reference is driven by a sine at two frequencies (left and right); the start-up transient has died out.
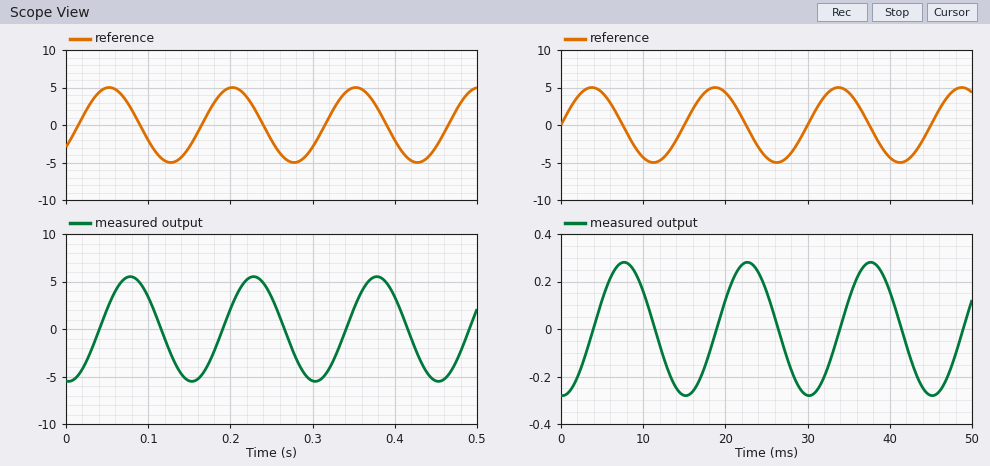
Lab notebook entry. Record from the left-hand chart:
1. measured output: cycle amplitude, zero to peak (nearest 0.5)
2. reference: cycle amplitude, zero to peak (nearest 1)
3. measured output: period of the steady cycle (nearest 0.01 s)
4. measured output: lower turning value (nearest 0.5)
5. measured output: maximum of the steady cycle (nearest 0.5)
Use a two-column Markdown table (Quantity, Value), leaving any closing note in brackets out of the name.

| Quantity | Value |
|---|---|
| measured output: cycle amplitude, zero to peak | 5.5 |
| reference: cycle amplitude, zero to peak | 5 |
| measured output: period of the steady cycle | 0.15 s |
| measured output: lower turning value | -5.5 |
| measured output: maximum of the steady cycle | 5.5 |
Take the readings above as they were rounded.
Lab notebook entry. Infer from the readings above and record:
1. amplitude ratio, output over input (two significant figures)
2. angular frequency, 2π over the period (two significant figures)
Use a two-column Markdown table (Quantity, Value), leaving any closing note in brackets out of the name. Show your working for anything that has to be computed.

| Quantity | Value |
|---|---|
| amplitude ratio, output over input | 5.5 / 5 = 1.1 |
| angular frequency, 2π over the period | 2π / 0.15 = 42 rad/s |
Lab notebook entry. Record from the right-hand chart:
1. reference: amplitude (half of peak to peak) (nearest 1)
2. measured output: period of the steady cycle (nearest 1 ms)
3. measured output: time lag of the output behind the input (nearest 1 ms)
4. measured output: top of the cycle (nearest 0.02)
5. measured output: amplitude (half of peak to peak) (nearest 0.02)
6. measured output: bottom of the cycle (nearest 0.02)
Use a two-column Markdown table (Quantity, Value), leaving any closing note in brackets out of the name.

| Quantity | Value |
|---|---|
| reference: amplitude (half of peak to peak) | 5 |
| measured output: period of the steady cycle | 15 ms |
| measured output: time lag of the output behind the input | 4 ms |
| measured output: top of the cycle | 0.28 |
| measured output: amplitude (half of peak to peak) | 0.28 |
| measured output: bottom of the cycle | -0.28 |
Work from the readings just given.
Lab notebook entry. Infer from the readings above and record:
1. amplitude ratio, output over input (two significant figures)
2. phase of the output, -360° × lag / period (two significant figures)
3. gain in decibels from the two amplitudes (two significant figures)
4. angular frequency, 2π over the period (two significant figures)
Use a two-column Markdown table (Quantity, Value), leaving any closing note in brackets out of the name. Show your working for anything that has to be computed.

| Quantity | Value |
|---|---|
| amplitude ratio, output over input | 0.28 / 5 = 0.056 |
| phase of the output, -360° × lag / period | -360 × 4 / 15 = -96° |
| gain in decibels from the two amplitudes | 20 log10(0.28 / 5) = -25 dB |
| angular frequency, 2π over the period | 2π / 15 = 0.42 rad/ms |
